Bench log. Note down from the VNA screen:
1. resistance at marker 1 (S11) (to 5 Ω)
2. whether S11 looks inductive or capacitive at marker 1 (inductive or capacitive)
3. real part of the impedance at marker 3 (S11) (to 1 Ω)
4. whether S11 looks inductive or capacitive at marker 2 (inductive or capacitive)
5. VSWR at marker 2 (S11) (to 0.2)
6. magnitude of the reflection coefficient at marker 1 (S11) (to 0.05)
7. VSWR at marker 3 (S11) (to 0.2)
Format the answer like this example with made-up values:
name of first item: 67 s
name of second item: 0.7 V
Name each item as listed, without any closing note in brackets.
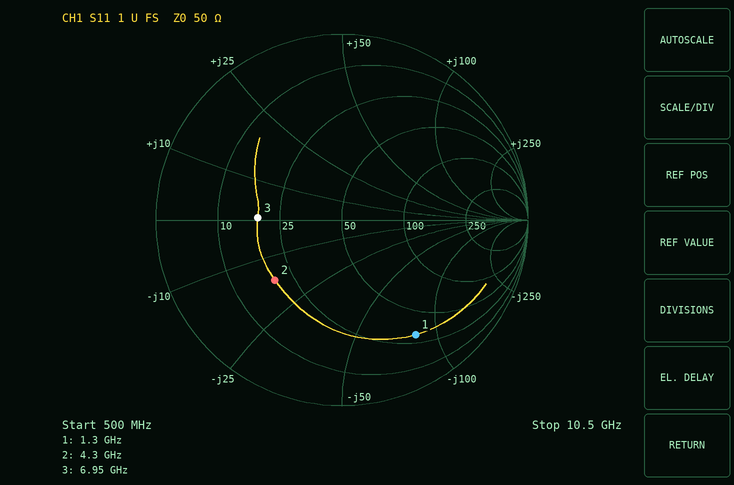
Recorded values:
resistance at marker 1 (S11): 30 Ω
whether S11 looks inductive or capacitive at marker 1: capacitive
real part of the impedance at marker 3 (S11): 19 Ω
whether S11 looks inductive or capacitive at marker 2: capacitive
VSWR at marker 2 (S11): 2.8
magnitude of the reflection coefficient at marker 1 (S11): 0.75
VSWR at marker 3 (S11): 2.6
